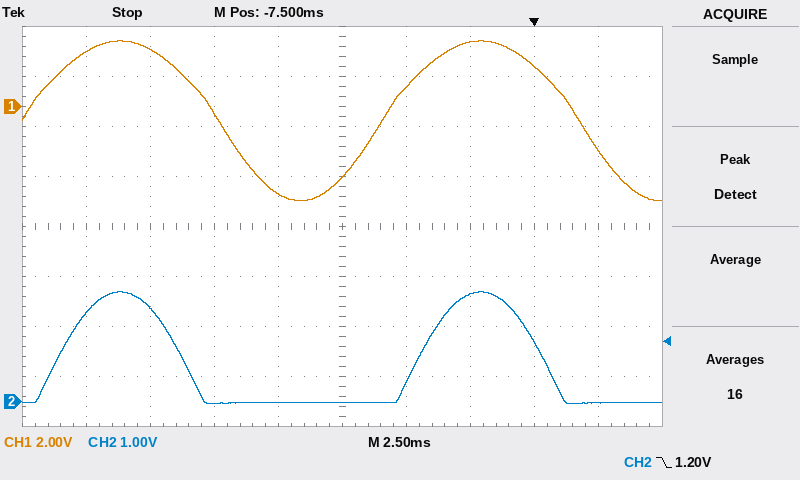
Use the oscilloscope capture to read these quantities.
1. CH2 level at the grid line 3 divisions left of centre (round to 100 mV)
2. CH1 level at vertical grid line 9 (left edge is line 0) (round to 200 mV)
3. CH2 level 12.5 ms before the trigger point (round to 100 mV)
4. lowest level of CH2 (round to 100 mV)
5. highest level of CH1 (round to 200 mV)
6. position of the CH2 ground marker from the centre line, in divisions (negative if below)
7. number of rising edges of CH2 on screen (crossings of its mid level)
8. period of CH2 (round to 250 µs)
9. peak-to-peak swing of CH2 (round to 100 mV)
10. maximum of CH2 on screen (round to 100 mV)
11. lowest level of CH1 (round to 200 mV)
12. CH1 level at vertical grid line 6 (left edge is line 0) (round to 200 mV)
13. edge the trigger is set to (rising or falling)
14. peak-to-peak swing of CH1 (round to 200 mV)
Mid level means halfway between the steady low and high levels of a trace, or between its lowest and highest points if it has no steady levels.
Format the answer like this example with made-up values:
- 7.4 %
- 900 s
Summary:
- 1.9 V
- -1.8 V
- 0.0 V
- 0.0 V
- 2.6 V
- -3.5 div
- 2
- 14.00 ms
- 2.2 V
- 2.2 V
- -3.8 V
- 800 mV
- falling
- 6.4 V
